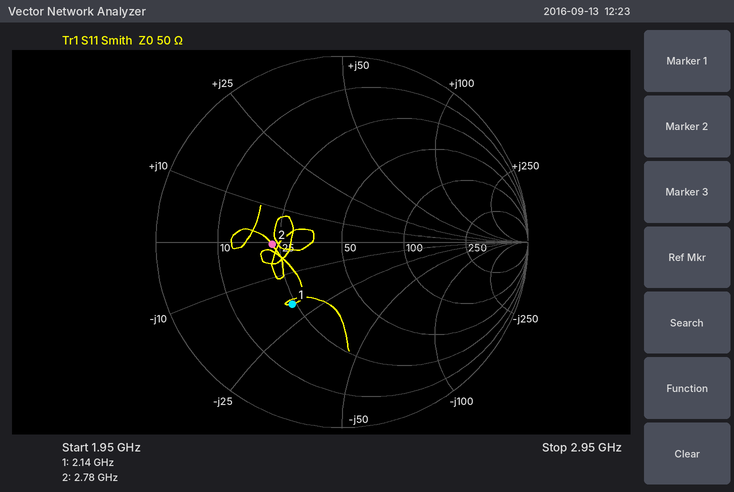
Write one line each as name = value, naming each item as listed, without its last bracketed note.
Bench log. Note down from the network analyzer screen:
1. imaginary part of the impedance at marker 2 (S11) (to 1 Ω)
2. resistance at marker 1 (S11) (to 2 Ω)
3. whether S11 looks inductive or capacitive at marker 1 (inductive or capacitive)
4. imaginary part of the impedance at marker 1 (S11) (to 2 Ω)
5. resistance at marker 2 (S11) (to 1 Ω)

imaginary part of the impedance at marker 2 (S11) = -1 Ω
resistance at marker 1 (S11) = 24 Ω
whether S11 looks inductive or capacitive at marker 1 = capacitive
imaginary part of the impedance at marker 1 (S11) = -20 Ω
resistance at marker 2 (S11) = 23 Ω
